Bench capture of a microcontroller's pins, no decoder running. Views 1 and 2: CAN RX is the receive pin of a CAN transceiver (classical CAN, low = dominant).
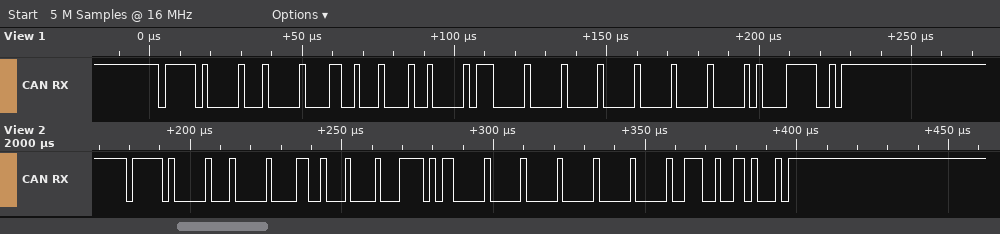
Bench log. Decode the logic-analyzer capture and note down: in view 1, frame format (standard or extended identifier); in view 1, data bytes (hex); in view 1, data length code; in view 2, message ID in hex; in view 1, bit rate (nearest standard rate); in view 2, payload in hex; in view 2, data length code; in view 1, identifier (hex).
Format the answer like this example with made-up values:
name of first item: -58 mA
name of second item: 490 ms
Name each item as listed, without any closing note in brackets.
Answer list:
in view 1, frame format: standard
in view 1, data bytes: 03 22 12 07 00 00 00 00
in view 1, data length code: 8
in view 2, message ID in hex: 0x7E0
in view 1, bit rate: 500 kbit/s
in view 2, payload in hex: 03 22 11 EB 00 00 00 00
in view 2, data length code: 8
in view 1, identifier: 0x7E0
